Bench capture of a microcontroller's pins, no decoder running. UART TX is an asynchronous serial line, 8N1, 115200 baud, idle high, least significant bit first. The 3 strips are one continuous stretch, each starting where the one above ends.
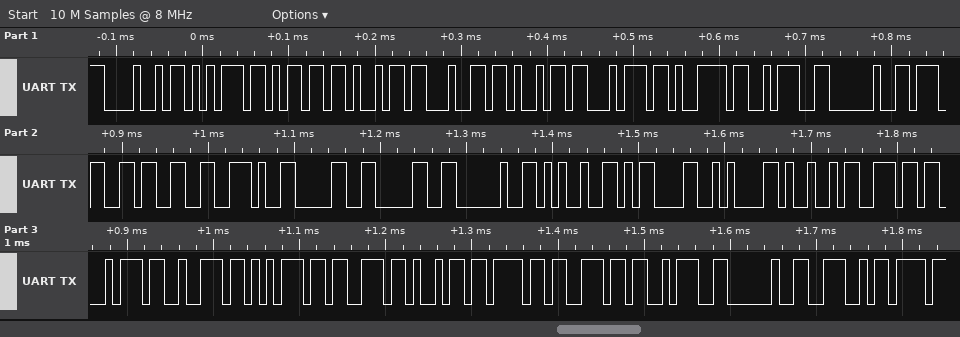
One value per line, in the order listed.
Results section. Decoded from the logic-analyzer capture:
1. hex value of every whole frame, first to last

48 75 6D 69 64 69 74 79 3A 20 37 33 2E 30 30 20 25 0D 0A 49 6E 74 72 75 73 69 6F 6E 3A 20 4E
